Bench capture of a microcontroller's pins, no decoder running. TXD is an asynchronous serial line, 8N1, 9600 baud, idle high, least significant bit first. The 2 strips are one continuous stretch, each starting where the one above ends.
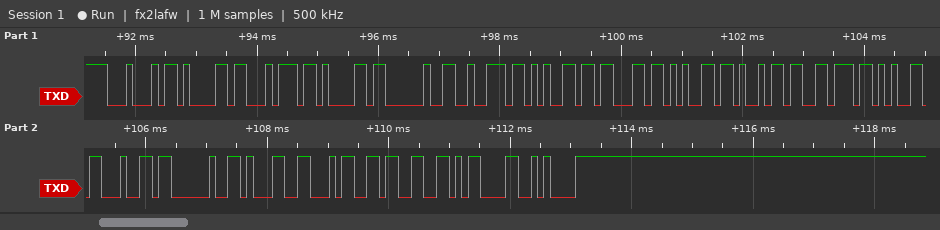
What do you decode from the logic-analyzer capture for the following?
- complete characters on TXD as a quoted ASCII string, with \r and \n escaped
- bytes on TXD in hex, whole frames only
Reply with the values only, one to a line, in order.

"Data received 143\r\n"
44 61 74 61 20 72 65 63 65 69 76 65 64 20 31 34 33 0D 0A
